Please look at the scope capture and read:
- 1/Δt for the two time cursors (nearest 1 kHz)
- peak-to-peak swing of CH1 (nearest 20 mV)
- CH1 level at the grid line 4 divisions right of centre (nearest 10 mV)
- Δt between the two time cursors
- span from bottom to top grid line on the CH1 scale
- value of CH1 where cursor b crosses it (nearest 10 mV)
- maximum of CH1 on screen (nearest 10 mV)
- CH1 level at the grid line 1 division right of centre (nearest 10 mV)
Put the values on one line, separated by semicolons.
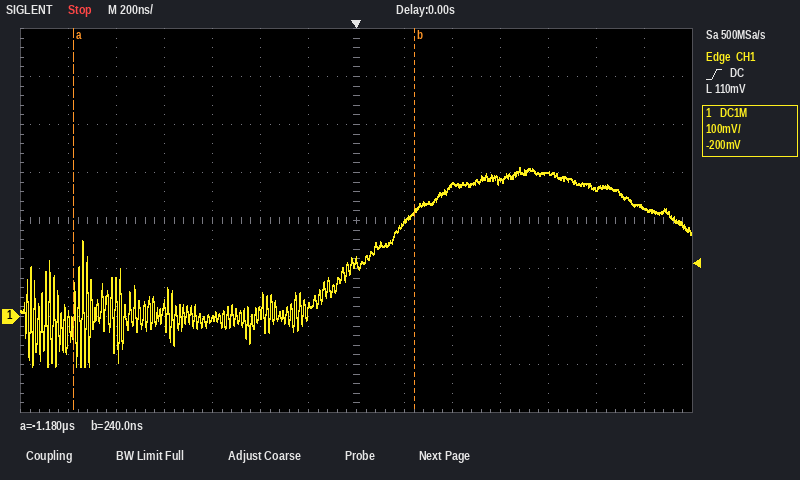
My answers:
704 kHz; 420 mV; 300 mV; 1.42 µs; 800 mV; 220 mV; 310 mV; 200 mV
